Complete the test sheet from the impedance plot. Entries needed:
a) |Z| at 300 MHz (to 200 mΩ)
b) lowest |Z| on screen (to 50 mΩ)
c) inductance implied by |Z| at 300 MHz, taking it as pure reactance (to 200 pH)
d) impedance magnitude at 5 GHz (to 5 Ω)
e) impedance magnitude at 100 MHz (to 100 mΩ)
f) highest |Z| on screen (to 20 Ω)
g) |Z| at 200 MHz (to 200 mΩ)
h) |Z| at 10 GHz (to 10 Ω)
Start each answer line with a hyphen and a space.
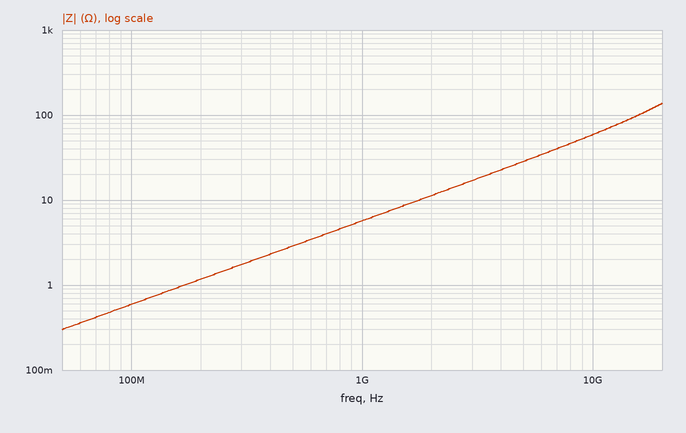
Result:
- 1.8 Ω
- 300 mΩ
- 1.0 nH
- 30 Ω
- 600 mΩ
- 140 Ω
- 1.2 Ω
- 60 Ω
